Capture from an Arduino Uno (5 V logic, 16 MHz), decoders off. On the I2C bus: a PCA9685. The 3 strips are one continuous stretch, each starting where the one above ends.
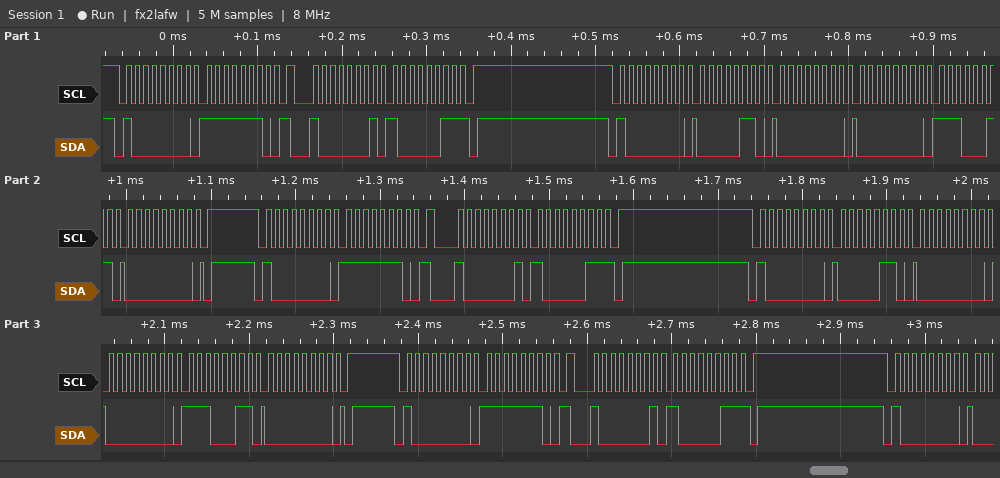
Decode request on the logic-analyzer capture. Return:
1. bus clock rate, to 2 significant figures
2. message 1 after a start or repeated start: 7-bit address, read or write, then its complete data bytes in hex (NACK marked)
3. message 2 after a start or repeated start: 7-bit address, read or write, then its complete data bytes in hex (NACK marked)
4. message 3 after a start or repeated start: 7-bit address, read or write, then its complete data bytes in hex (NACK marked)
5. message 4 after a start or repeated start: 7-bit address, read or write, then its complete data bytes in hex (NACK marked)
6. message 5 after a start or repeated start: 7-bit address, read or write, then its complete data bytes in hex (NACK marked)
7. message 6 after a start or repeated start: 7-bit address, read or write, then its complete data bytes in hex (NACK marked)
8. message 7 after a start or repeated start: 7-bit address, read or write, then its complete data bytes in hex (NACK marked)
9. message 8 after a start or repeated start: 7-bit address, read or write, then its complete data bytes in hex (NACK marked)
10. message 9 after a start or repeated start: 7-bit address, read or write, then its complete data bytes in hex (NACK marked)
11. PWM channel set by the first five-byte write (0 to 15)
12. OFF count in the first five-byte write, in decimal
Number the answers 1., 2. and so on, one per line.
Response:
1. 100 kHz
2. 0x40 write: FE
3. 0x40 read: 83 NACK
4. 0x40 write: 06 00 00 E3 00
5. 0x40 write: FE
6. 0x40 read: 83 NACK
7. 0x40 write: 06 00 00 E3 00
8. 0x40 write: FE
9. 0x40 read: 83 NACK
10. 0x40 write
11. 0
12. 227
